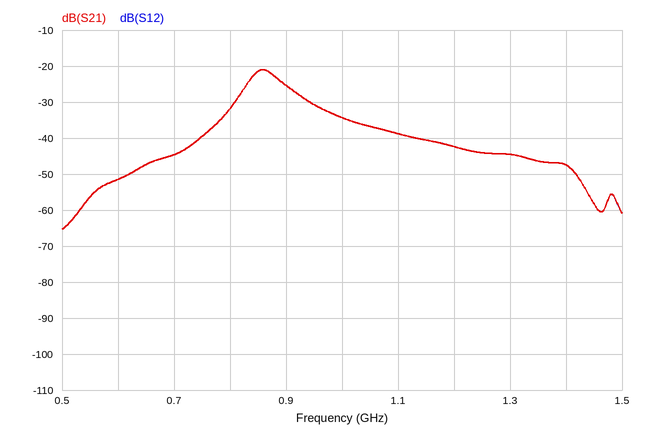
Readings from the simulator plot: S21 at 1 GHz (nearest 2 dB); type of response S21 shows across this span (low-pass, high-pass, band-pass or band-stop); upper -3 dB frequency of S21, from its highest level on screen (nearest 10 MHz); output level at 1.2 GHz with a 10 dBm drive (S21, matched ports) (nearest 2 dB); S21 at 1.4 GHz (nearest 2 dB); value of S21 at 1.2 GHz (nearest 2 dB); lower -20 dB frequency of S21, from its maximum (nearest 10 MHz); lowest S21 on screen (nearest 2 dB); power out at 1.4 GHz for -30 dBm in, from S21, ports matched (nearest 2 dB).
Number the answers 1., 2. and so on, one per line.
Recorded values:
1. -34 dB
2. band-pass
3. 890 MHz
4. -32 dBm
5. -48 dB
6. -42 dB
7. 740 MHz
8. -66 dB
9. -78 dBm
